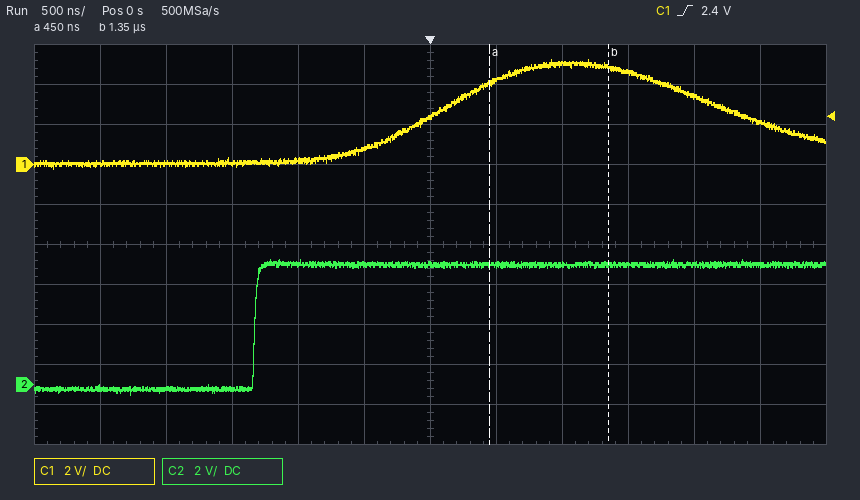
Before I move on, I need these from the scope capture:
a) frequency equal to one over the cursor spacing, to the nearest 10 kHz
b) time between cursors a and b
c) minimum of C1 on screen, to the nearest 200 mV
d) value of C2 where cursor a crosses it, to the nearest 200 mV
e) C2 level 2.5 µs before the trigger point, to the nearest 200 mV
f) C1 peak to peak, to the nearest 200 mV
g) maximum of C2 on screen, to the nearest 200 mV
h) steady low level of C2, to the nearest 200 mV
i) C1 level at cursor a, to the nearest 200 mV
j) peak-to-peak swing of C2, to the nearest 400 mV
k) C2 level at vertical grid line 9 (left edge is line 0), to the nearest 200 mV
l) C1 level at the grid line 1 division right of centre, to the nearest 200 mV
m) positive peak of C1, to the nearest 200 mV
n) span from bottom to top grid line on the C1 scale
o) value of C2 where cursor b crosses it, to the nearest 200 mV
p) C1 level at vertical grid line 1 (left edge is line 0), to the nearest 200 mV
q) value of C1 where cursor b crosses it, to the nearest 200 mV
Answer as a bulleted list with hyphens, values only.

- 1.11 MHz
- 900 ns
- -200 mV
- 6.0 V
- -200 mV
- 5.4 V
- 6.2 V
- -200 mV
- 4.2 V
- 6.8 V
- 6.0 V
- 4.2 V
- 5.2 V
- 20 V
- 6.0 V
- 0.0 V
- 4.8 V
